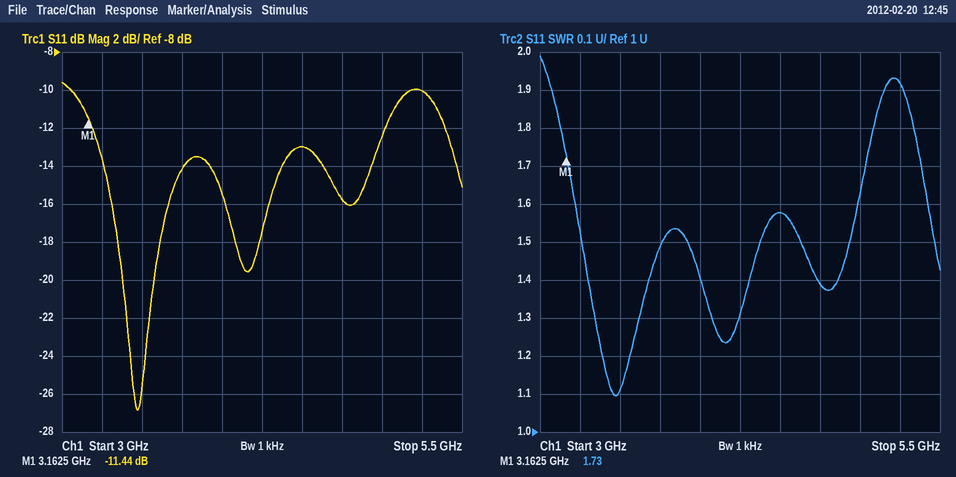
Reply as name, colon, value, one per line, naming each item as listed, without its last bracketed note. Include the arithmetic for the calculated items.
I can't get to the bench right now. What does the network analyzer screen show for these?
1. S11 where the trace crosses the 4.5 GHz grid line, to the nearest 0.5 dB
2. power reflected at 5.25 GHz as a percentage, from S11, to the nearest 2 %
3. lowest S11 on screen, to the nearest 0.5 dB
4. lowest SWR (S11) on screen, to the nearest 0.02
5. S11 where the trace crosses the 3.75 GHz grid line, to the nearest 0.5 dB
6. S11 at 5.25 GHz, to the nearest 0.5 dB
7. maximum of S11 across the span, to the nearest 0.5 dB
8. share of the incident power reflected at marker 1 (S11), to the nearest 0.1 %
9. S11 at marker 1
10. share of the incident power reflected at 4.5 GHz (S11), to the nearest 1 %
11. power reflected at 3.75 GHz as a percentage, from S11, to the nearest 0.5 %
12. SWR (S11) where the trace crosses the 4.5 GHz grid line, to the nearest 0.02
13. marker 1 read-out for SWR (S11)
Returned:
S11 where the trace crosses the 4.5 GHz grid line, to the nearest 0.5 dB: -13.0 dB
power reflected at 5.25 GHz as a percentage, from S11, to the nearest 2 %: 10^(-10/10) ≈ 10 %
lowest S11 on screen, to the nearest 0.5 dB: -27.0 dB
lowest SWR (S11) on screen, to the nearest 0.02: 1.10
S11 where the trace crosses the 3.75 GHz grid line, to the nearest 0.5 dB: -14.0 dB
S11 at 5.25 GHz, to the nearest 0.5 dB: -10.0 dB
maximum of S11 across the span, to the nearest 0.5 dB: -9.5 dB
share of the incident power reflected at marker 1 (S11), to the nearest 0.1 %: 10^(-11.44/10) ≈ 7.2 %
S11 at marker 1: -11.44 dB
share of the incident power reflected at 4.5 GHz (S11), to the nearest 1 %: 10^(-13/10) ≈ 5 %
power reflected at 3.75 GHz as a percentage, from S11, to the nearest 0.5 %: 10^(-14/10) ≈ 4.0 %
SWR (S11) where the trace crosses the 4.5 GHz grid line, to the nearest 0.02: 1.58
marker 1 read-out for SWR: 1.73
